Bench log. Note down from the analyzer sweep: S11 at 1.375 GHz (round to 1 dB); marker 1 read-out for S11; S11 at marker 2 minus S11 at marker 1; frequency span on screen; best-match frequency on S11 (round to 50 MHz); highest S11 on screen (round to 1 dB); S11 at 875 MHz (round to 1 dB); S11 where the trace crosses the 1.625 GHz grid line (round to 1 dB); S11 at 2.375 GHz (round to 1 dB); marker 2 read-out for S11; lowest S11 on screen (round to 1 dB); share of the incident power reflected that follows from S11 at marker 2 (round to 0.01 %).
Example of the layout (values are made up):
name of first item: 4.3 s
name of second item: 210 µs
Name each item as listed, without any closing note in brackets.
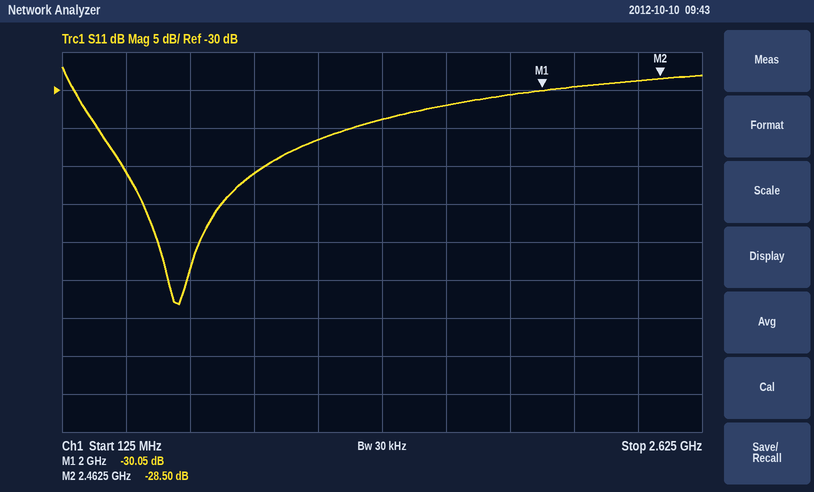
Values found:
S11 at 1.375 GHz: -34 dB
marker 1 read-out for S11: -30.05 dB
S11 at marker 2 minus S11 at marker 1: 1.55 dB
frequency span on screen: 2.5 GHz
best-match frequency on S11: 600 MHz
highest S11 on screen: -27 dB
S11 at 875 MHz: -41 dB
S11 where the trace crosses the 1.625 GHz grid line: -32 dB
S11 at 2.375 GHz: -29 dB
marker 2 read-out for S11: -28.50 dB
lowest S11 on screen: -58 dB
share of the incident power reflected that follows from S11 at marker 2: 0.14 %
